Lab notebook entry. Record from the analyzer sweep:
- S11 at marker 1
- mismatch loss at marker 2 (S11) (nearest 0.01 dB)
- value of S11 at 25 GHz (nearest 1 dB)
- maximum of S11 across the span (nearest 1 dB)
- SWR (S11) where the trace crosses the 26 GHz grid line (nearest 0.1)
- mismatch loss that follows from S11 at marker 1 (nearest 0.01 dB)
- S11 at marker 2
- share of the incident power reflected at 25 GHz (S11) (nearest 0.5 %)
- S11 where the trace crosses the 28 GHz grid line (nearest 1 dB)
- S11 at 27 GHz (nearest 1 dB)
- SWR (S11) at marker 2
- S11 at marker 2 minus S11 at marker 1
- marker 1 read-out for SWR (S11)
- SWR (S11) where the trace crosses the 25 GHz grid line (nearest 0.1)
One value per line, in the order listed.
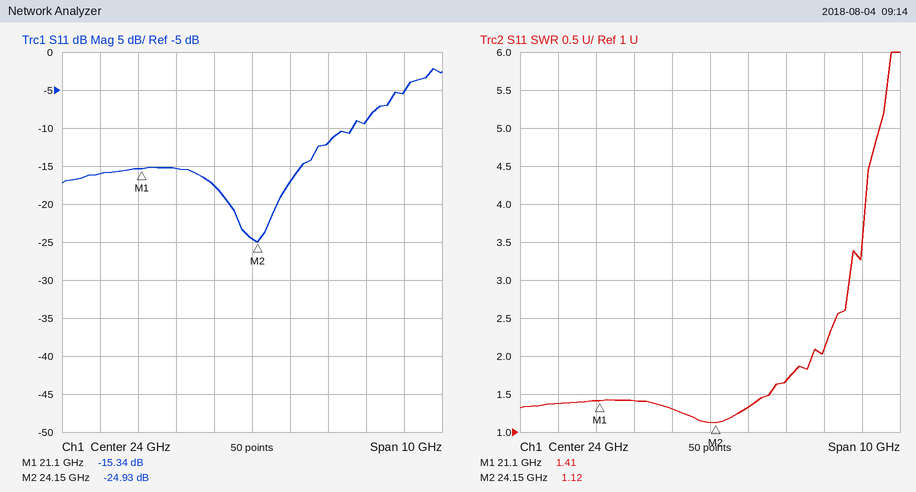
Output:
-15.34 dB
0.01 dB
-17 dB
-2 dB
1.7
0.13 dB
-24.93 dB
2.0 %
-5 dB
-9 dB
1.12
-9.59 dB
1.41
1.3
